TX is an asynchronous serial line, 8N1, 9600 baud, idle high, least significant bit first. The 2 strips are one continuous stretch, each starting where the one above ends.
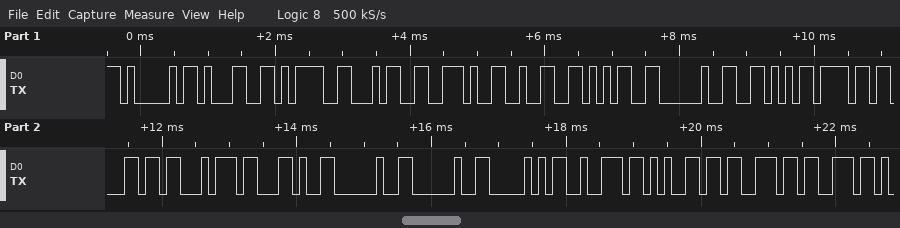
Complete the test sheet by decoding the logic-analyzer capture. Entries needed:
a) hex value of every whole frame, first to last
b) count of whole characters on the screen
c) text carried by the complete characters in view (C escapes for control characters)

41 31 3D 34 2E 32 35 20 56 6F 6C 74 2C 20 20 50 72 65 73 73
20
"A1=4.25 Volt,  Press"
